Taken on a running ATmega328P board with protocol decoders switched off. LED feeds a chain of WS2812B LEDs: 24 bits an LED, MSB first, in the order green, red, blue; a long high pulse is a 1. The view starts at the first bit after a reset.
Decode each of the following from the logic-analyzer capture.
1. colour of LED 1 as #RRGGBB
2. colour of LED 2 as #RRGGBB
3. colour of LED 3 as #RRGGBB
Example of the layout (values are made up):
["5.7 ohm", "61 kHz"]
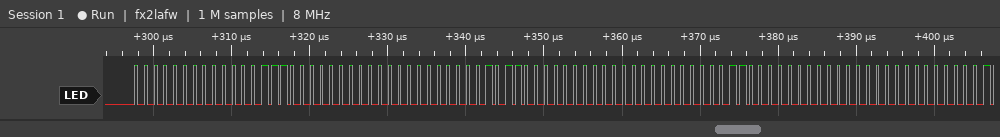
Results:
["#070000", "#0B0000", "#060000"]
